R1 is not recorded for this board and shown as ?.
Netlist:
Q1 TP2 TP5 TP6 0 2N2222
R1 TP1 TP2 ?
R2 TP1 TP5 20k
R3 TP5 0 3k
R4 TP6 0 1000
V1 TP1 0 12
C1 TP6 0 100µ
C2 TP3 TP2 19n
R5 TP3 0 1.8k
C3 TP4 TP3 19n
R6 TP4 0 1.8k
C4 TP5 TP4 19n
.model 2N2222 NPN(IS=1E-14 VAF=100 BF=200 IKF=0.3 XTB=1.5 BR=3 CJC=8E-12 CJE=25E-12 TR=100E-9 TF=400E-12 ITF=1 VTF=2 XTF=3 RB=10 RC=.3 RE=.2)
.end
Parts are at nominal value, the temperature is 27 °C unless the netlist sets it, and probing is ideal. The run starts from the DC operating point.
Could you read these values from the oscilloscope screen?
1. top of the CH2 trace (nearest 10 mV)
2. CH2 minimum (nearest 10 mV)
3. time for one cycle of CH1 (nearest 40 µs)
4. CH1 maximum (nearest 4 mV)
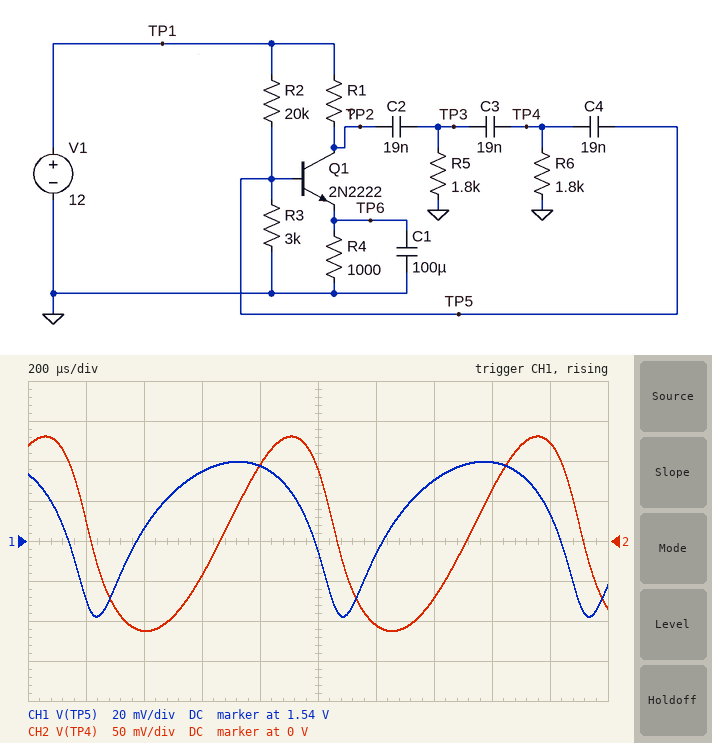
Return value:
130 mV
-110 mV
840 µs
1.580 V
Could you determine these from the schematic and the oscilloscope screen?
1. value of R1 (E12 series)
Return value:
3.9 kΩ
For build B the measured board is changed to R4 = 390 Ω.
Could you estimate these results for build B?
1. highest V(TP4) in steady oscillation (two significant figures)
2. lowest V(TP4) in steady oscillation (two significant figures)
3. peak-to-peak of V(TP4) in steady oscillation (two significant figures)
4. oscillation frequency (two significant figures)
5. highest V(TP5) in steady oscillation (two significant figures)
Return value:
150 mV
-160 mV
310 mV
1.3 kHz
1.5 V
